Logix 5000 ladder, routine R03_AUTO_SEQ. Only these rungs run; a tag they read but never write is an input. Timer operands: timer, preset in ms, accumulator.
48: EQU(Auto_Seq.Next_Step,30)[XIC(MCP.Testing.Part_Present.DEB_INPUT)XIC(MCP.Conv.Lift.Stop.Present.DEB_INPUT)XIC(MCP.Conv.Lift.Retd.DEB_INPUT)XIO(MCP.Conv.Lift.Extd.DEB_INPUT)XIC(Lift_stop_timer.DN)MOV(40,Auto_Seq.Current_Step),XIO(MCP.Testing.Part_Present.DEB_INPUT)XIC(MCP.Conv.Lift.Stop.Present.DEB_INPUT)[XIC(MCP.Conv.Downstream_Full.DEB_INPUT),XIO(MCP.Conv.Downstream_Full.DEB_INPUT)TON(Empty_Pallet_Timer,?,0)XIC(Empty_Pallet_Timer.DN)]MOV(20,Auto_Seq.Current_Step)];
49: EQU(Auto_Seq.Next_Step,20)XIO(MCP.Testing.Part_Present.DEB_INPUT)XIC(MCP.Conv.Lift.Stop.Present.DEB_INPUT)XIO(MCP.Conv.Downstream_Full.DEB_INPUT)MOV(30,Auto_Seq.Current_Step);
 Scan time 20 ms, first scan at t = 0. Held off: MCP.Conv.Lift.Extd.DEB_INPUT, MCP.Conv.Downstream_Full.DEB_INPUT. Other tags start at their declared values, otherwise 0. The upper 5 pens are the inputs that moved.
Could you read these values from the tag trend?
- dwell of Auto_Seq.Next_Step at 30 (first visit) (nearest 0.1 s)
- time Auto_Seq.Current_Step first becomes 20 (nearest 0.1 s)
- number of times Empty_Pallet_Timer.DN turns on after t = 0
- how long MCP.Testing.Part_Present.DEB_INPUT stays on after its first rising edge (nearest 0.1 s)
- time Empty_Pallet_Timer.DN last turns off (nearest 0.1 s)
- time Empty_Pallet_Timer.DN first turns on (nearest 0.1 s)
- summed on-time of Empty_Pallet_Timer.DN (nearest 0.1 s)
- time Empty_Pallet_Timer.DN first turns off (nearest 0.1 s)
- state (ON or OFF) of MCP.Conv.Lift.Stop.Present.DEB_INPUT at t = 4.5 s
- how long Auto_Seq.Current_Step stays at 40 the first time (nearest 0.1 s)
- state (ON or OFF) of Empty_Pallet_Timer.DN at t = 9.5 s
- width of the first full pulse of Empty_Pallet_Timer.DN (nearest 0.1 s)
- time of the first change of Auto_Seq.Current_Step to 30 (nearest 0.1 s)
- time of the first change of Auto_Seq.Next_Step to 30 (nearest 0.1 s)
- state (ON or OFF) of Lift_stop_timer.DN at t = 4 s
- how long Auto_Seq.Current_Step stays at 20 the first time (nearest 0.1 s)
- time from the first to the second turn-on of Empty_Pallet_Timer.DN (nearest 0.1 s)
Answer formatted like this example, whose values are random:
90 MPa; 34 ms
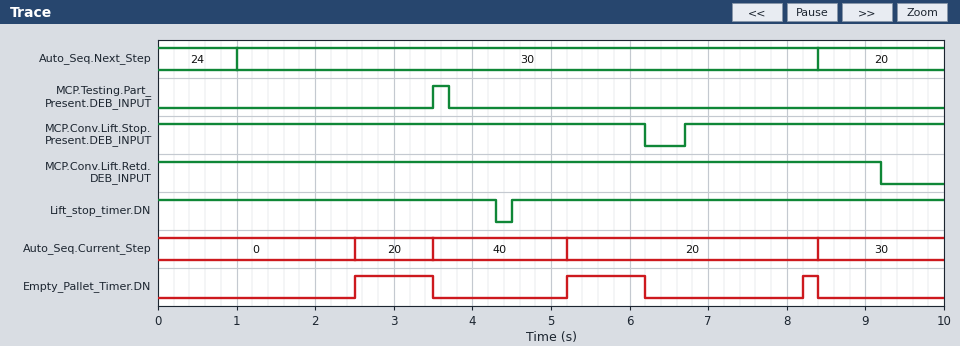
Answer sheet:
7.4 s; 2.5 s; 3; 0.2 s; 8.4 s; 2.5 s; 2.2 s; 3.5 s; ON; 1.7 s; OFF; 1.0 s; 8.4 s; 1.0 s; ON; 1.0 s; 2.7 s
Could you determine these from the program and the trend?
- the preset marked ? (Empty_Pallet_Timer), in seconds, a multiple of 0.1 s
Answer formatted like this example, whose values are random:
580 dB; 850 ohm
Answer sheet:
1.5 s
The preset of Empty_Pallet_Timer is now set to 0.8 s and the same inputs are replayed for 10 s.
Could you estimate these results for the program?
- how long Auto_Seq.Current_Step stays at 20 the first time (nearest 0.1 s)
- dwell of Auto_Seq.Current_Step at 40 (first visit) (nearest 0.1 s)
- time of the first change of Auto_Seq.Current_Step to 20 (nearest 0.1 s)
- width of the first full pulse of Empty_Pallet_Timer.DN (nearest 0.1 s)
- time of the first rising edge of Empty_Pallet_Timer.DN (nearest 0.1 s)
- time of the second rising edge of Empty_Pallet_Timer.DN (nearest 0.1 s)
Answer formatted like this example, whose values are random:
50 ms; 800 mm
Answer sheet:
1.7 s; 1.0 s; 1.8 s; 1.7 s; 1.8 s; 4.5 s
